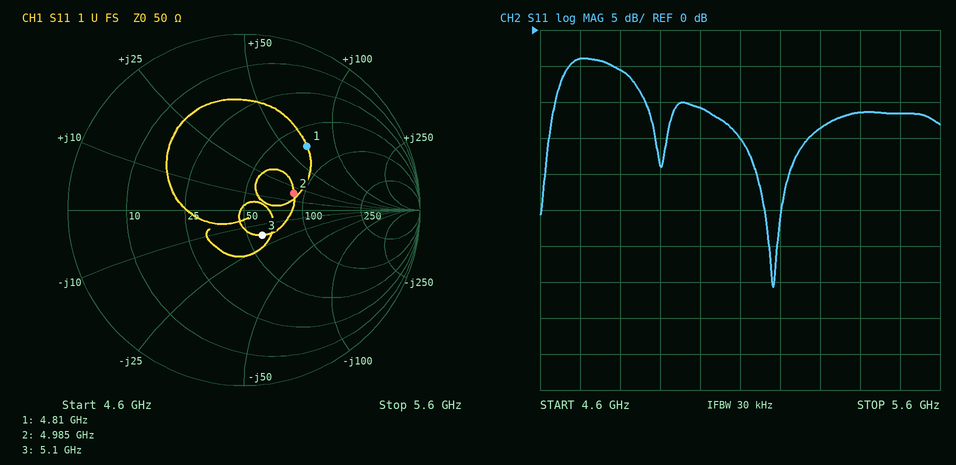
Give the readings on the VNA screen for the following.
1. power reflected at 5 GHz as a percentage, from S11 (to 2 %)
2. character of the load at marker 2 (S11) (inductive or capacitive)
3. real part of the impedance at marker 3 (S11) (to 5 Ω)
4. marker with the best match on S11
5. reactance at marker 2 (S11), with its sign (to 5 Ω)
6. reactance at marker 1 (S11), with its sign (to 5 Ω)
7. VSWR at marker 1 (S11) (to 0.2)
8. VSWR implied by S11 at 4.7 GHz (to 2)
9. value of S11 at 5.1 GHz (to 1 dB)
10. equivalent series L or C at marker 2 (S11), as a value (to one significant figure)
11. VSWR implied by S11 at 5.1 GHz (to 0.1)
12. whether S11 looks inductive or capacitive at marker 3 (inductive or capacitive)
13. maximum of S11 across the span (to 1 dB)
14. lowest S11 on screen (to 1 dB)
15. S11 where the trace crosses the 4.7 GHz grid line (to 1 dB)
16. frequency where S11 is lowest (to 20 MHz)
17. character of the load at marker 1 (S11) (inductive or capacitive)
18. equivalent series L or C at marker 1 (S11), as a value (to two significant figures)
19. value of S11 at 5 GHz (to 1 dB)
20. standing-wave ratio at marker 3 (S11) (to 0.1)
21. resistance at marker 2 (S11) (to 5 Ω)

8 %
inductive
60 Ω
marker 3
+20 Ω
+65 Ω
3.0
4
-15 dB
600 pH
1.4
capacitive
-4 dB
-36 dB
-4 dB
5.18 GHz
inductive
2.2 nH
-11 dB
1.4
85 Ω
